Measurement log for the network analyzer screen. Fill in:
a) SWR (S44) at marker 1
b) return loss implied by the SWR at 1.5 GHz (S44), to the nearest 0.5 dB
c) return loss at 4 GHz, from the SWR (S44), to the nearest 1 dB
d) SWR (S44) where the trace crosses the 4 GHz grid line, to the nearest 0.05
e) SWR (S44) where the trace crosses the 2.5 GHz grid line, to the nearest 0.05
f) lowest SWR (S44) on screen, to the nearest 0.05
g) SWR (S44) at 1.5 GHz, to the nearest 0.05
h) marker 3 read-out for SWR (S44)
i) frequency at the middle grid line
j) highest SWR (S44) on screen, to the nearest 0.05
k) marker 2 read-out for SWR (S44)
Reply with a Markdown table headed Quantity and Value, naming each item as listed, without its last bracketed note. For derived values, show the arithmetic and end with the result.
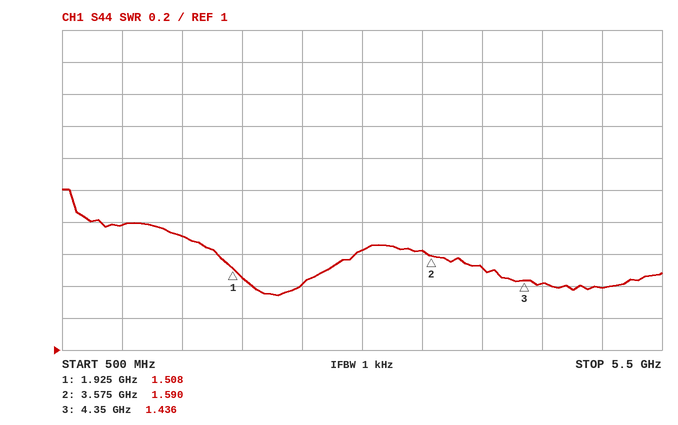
| Quantity | Value |
|---|---|
| SWR (S44) at marker 1 | 1.508 |
| return loss implied by the SWR at 1.5 GHz (S44), to the nearest 0.5 dB | −20 log10((1.7 − 1)/(1.7 + 1)) ≈ 11.7 dB, so 11.5 dB to the nearest 0.5 dB |
| return loss at 4 GHz, from the SWR (S44), to the nearest 1 dB | −20 log10((1.5 − 1)/(1.5 + 1)) ≈ 14 dB |
| SWR (S44) where the trace crosses the 4 GHz grid line, to the nearest 0.05 | 1.50 |
| SWR (S44) where the trace crosses the 2.5 GHz grid line, to the nearest 0.05 | 1.40 |
| lowest SWR (S44) on screen, to the nearest 0.05 | 1.35 |
| SWR (S44) at 1.5 GHz, to the nearest 0.05 | 1.70 |
| marker 3 read-out for SWR | 1.436 |
| frequency at the middle grid line | 3 GHz |
| highest SWR (S44) on screen, to the nearest 0.05 | 2.00 |
| marker 2 read-out for SWR | 1.590 |
